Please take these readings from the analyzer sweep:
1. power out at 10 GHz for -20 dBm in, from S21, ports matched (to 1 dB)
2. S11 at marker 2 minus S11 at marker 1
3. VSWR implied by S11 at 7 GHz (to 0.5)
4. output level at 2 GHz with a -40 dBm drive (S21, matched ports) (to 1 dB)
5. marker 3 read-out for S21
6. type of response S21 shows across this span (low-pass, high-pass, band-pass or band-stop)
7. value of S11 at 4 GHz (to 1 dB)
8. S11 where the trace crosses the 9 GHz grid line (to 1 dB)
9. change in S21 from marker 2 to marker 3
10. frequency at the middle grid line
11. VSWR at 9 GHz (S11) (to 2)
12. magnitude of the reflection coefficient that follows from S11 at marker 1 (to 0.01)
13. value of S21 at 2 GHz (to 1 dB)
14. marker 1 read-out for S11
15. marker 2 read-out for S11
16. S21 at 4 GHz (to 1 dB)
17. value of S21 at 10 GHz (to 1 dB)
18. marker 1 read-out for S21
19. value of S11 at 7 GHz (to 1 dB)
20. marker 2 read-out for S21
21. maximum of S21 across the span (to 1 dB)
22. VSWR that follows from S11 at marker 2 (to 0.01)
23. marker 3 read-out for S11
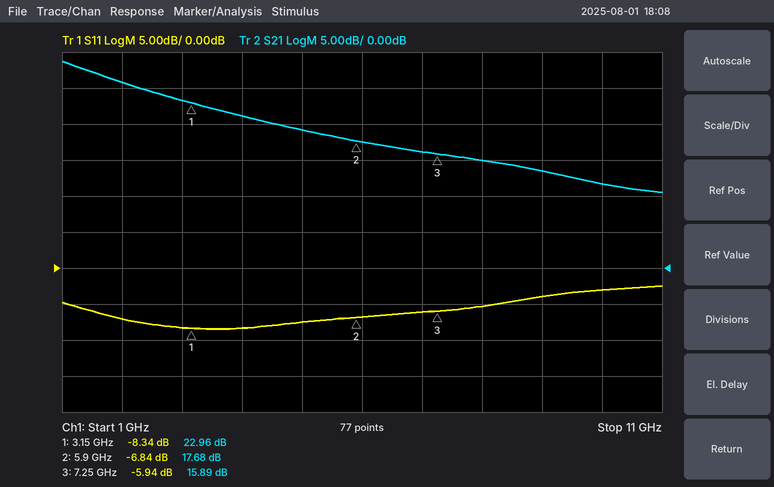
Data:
-8 dBm
1.50 dB
3.0
-14 dBm
15.89 dB
low-pass
-8 dB
-4 dB
-1.79 dB
6 GHz
4
0.38
26 dB
-8.34 dB
-6.84 dB
21 dB
12 dB
22.96 dB
-6 dB
17.68 dB
29 dB
2.67
-5.94 dB
